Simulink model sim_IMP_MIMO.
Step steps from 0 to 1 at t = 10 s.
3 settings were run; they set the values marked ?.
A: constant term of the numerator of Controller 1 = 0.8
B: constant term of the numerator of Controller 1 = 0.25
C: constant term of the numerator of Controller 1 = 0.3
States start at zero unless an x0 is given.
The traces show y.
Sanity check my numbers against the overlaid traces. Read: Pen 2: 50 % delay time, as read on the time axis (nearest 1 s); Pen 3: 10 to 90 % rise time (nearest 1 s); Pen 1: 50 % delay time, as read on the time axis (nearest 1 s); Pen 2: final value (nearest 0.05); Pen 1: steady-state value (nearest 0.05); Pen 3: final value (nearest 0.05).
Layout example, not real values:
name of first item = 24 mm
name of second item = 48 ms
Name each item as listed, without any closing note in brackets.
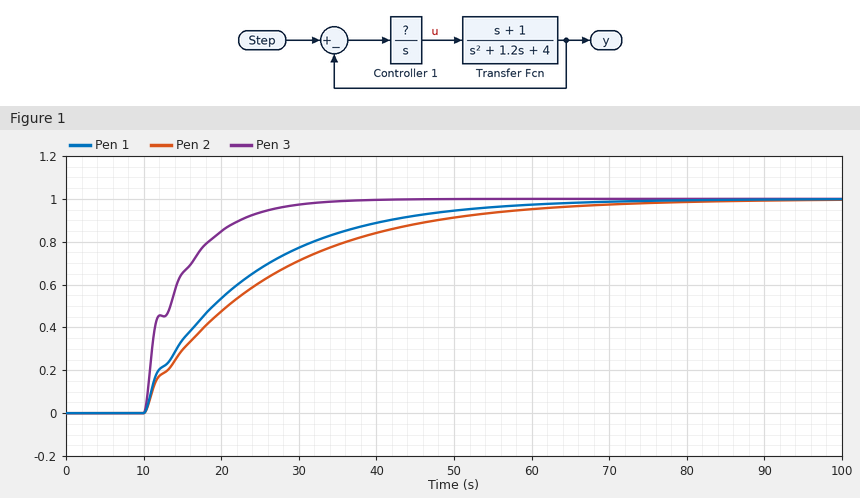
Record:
Pen 2: 50 % delay time, as read on the time axis = 21 s
Pen 3: 10 to 90 % rise time = 12 s
Pen 1: 50 % delay time, as read on the time axis = 19 s
Pen 2: final value = 1.00
Pen 1: steady-state value = 1.00
Pen 3: final value = 1.00
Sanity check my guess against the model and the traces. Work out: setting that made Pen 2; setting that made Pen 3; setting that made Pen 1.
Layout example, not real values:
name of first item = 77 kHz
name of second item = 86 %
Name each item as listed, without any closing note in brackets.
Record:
setting that made Pen 2 = B
setting that made Pen 3 = A
setting that made Pen 1 = C
